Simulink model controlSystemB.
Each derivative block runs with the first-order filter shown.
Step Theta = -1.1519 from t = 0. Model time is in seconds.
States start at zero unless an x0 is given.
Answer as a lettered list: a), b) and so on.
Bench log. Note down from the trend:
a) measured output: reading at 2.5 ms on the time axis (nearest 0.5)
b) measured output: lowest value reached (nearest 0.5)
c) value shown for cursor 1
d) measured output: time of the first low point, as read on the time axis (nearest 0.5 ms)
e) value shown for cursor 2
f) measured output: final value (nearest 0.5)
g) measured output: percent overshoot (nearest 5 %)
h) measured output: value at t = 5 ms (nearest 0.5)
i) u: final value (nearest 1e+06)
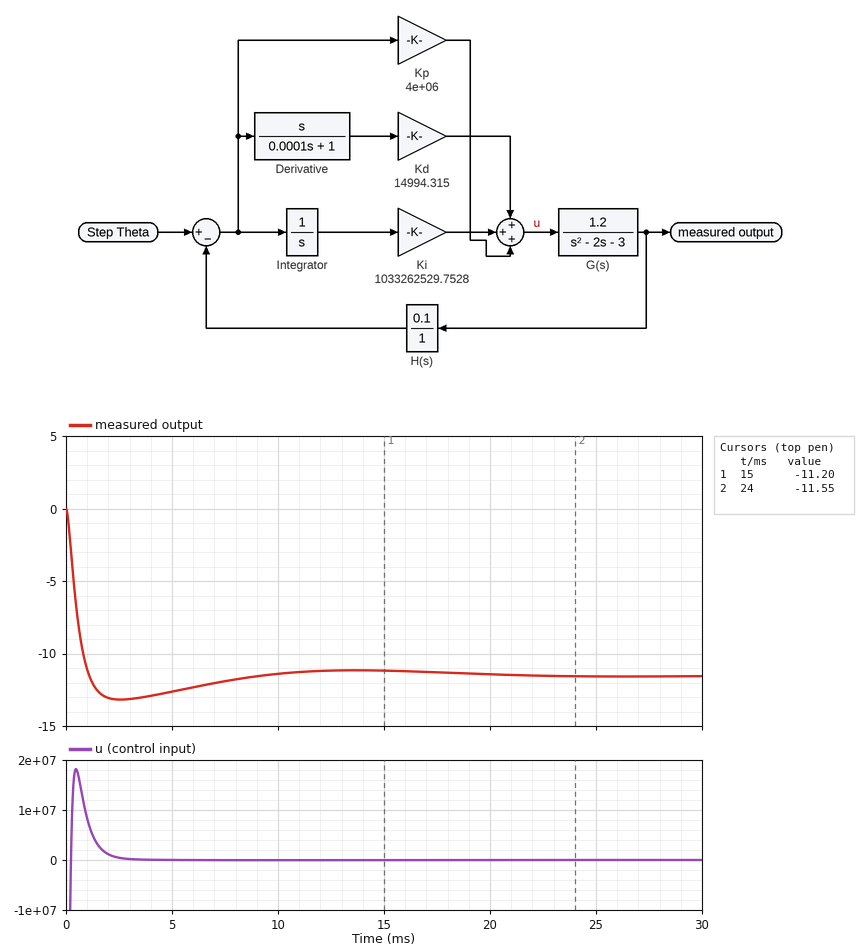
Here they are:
a) -13.0
b) -13.0
c) -11.20
d) 2.5 ms
e) -11.55
f) -11.5
g) 15 %
h) -12.5
i) 0
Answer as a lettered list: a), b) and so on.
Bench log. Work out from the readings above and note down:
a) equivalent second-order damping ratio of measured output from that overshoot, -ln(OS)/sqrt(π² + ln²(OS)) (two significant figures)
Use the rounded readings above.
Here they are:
a) 0.52
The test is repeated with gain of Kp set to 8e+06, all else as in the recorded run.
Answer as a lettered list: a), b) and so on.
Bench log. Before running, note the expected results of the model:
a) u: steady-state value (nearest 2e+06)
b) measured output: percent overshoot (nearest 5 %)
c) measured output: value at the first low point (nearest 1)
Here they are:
a) 0
b) 20 %
c) -14
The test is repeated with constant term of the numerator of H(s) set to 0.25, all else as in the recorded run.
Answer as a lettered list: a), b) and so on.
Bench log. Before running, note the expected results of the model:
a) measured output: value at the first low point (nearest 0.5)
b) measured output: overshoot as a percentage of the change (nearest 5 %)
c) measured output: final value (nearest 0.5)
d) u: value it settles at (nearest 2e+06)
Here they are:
a) -5.0
b) 10 %
c) -4.5
d) 0
